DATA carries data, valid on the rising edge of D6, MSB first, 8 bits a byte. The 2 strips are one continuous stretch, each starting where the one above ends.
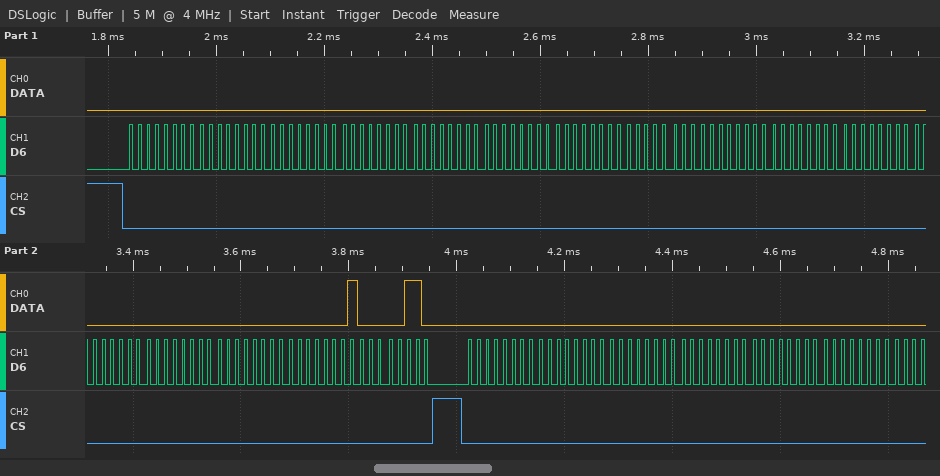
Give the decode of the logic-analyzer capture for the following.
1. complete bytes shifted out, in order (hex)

00 00 00 00 00 00 00 00 00 00 00 00 00 00 01 06 00 00 00 00 00 00
